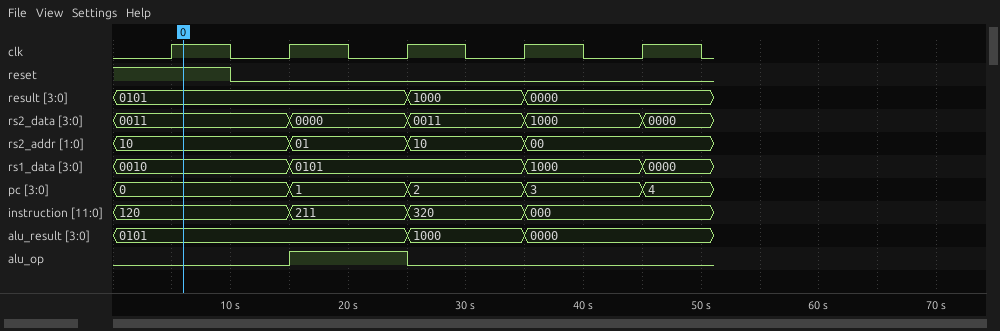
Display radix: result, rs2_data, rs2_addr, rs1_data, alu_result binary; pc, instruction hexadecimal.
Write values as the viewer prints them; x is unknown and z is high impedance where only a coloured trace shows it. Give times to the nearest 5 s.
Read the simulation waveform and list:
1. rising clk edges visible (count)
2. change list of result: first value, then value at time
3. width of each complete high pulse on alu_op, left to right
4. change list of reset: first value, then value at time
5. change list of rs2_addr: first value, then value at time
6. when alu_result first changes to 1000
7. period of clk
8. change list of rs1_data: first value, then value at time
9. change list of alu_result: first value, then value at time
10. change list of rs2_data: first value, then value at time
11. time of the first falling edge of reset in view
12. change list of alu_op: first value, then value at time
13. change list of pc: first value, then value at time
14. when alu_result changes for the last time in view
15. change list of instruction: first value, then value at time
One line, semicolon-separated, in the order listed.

5; 0101, 1000 at 25 s, 0000 at 35 s; 10 s; 1, 0 at 10 s; 10, 01 at 15 s, 10 at 25 s, 00 at 35 s; 25 s; 10 s; 0010, 0101 at 15 s, 1000 at 35 s, 0000 at 45 s; 0101, 1000 at 25 s, 0000 at 35 s; 0011, 0000 at 15 s, 0011 at 25 s, 1000 at 35 s, 0000 at 45 s; 10 s; 0, 1 at 15 s, 0 at 25 s; 0, 1 at 15 s, 2 at 25 s, 3 at 35 s, 4 at 45 s; 35 s; 120, 211 at 15 s, 320 at 25 s, 000 at 35 s
